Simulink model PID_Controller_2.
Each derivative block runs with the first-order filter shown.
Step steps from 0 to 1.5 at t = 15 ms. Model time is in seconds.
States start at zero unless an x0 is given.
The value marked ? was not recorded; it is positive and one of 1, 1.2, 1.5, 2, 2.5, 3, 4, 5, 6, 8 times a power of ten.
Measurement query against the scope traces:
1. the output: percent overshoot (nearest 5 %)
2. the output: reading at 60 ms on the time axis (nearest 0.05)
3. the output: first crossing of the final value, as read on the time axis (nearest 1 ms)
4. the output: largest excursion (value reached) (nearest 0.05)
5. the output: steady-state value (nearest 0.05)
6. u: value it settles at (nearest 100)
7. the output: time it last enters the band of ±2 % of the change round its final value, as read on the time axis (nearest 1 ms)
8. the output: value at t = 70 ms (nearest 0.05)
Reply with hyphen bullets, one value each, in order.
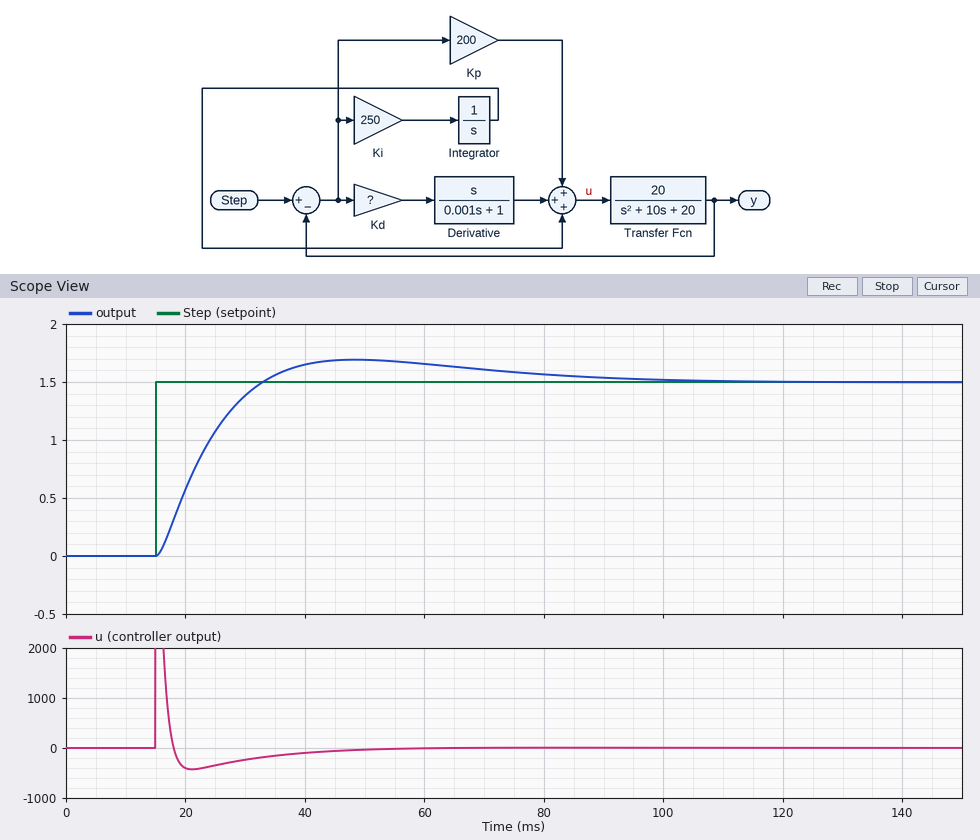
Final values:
- 15 %
- 1.65
- 33 ms
- 1.70
- 1.50
- 0
- 94 ms
- 1.60
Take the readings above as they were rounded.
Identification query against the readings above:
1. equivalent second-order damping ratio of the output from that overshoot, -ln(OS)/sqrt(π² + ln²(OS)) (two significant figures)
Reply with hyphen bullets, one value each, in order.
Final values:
- 0.52
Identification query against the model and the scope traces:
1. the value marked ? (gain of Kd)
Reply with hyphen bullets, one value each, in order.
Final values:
- 5
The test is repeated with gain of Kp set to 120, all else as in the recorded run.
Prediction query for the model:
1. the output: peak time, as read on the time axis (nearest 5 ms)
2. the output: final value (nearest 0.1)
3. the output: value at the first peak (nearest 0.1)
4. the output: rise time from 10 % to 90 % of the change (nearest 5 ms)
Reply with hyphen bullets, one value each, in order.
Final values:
- 55 ms
- 1.5
- 1.6
- 15 ms
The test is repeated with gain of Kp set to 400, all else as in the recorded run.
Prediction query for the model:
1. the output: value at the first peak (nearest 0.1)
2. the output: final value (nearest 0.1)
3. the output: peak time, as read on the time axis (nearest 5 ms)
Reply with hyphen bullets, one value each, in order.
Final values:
- 1.8
- 1.5
- 40 ms
